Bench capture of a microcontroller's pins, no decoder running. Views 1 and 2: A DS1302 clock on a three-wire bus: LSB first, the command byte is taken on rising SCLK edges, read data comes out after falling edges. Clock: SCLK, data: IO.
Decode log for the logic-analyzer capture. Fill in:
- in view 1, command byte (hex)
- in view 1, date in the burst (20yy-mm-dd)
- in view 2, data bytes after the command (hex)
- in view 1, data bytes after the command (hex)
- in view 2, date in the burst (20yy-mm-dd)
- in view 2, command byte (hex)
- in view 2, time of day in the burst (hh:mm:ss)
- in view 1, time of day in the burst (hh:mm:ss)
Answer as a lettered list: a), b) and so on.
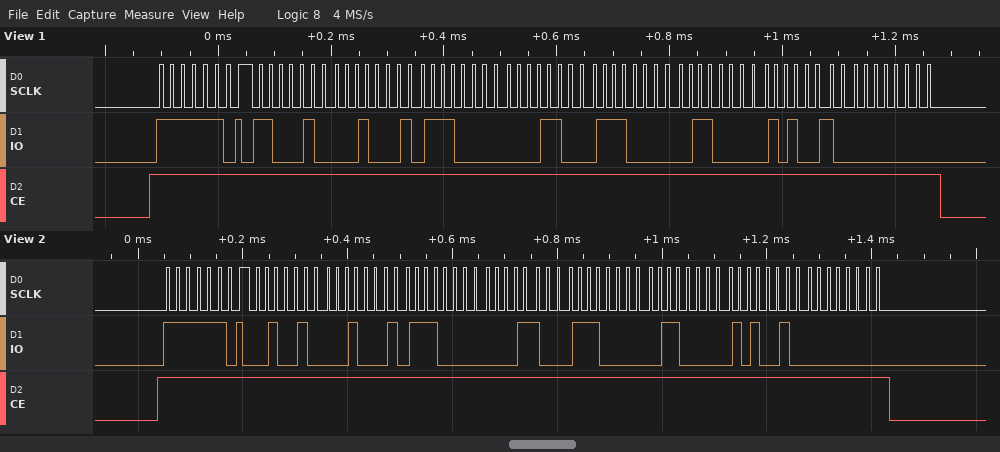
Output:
a) 0xBF
b) 2025-07-18
c) 24 44 07 18 07 06 25 00
d) 23 44 07 18 07 06 25 00
e) 2025-07-18
f) 0xBF
g) 07:44:24
h) 07:44:23
